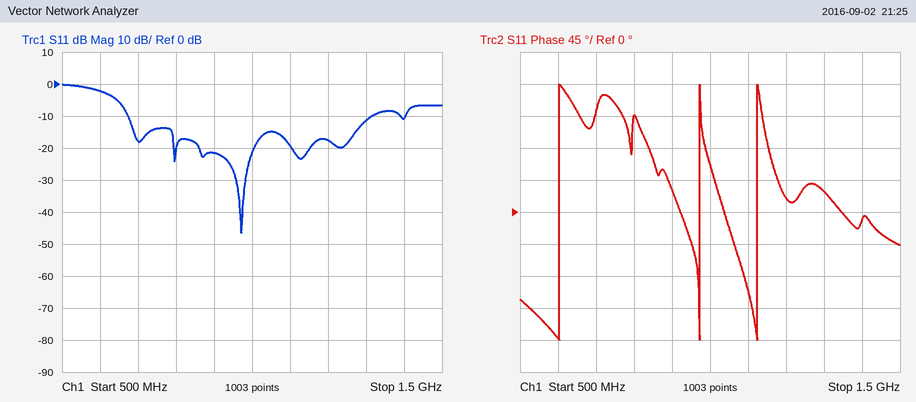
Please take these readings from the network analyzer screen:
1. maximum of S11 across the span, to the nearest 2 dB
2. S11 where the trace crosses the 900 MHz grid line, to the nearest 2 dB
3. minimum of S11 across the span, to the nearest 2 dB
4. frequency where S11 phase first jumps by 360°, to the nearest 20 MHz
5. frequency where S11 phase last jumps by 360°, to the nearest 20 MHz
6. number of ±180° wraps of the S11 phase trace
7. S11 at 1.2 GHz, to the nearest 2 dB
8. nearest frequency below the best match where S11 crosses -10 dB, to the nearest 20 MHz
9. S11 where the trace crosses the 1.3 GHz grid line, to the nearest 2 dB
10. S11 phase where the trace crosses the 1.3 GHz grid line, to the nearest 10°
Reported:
0 dB
-22 dB
-46 dB
600 MHz
1.12 GHz
3
-18 dB
680 MHz
-12 dB
30°
